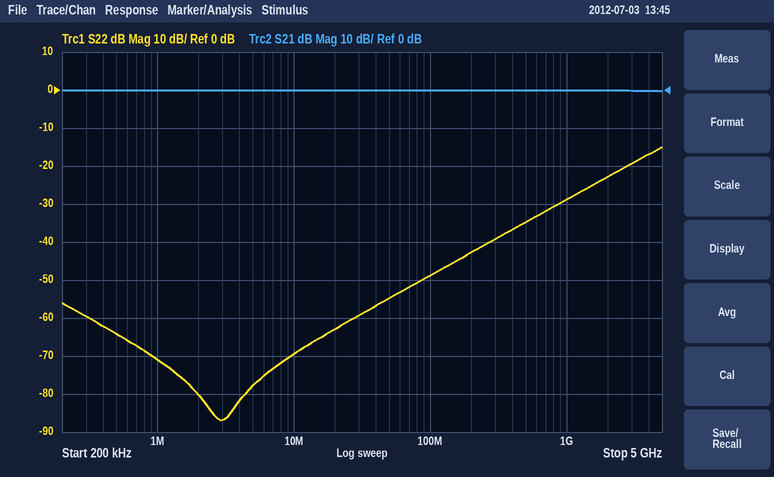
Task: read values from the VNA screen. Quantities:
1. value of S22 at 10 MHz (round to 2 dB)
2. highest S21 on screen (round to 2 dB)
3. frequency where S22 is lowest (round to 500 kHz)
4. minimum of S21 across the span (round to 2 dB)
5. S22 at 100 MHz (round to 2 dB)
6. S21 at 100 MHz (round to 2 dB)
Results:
-70 dB
0 dB
3.0 MHz
0 dB
-48 dB
0 dB
